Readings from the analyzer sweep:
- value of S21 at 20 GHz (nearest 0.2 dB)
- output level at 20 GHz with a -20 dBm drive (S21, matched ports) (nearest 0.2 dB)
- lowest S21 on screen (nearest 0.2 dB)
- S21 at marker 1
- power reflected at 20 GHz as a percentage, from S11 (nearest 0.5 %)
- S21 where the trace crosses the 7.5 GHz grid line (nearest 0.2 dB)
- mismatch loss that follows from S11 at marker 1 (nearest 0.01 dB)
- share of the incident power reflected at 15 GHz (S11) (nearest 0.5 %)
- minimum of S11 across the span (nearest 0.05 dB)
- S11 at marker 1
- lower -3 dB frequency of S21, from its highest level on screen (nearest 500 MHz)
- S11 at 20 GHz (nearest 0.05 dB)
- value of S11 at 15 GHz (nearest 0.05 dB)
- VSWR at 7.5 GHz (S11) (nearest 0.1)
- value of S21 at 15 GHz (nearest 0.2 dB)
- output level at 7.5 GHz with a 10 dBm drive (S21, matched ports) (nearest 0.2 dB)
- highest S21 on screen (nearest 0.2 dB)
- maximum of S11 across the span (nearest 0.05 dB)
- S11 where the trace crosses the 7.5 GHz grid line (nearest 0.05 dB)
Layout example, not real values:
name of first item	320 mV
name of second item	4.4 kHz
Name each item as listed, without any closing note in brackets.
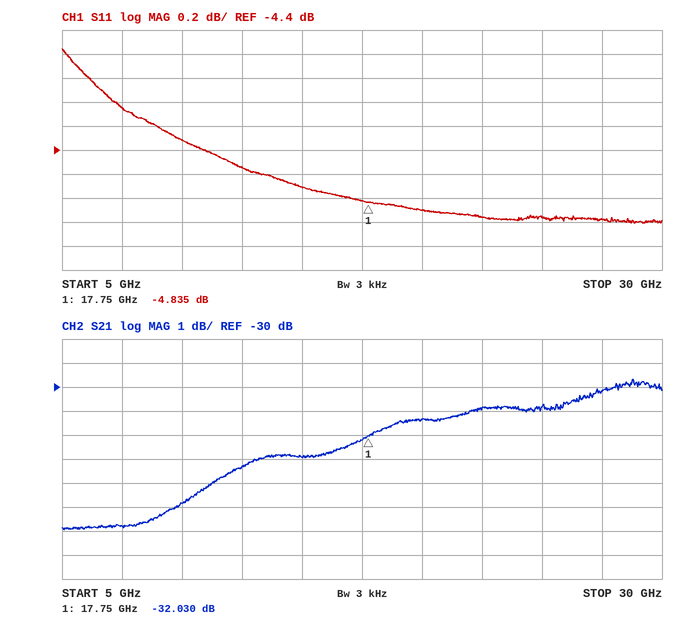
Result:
value of S21 at 20 GHz	-31.4 dB
output level at 20 GHz with a -20 dBm drive (S21, matched ports)	-51.4 dBm
lowest S21 on screen	-36.0 dB
S21 at marker 1	-32.030 dB
power reflected at 20 GHz as a percentage, from S11	32.5 %
S21 where the trace crosses the 7.5 GHz grid line	-35.8 dB
mismatch loss that follows from S11 at marker 1	1.73 dB
share of the incident power reflected at 15 GHz (S11)	34.0 %
minimum of S11 across the span	-5.00 dB
S11 at marker 1	-4.835 dB
lower -3 dB frequency of S21, from its highest level on screen	16.5 GHz
S11 at 20 GHz	-4.90 dB
value of S11 at 15 GHz	-4.70 dB
VSWR at 7.5 GHz (S11)	4.4
value of S21 at 15 GHz	-33.0 dB
output level at 7.5 GHz with a 10 dBm drive (S21, matched ports)	-25.8 dBm
highest S21 on screen	-29.6 dB
maximum of S11 across the span	-3.55 dB
S11 where the trace crosses the 7.5 GHz grid line	-4.05 dB
